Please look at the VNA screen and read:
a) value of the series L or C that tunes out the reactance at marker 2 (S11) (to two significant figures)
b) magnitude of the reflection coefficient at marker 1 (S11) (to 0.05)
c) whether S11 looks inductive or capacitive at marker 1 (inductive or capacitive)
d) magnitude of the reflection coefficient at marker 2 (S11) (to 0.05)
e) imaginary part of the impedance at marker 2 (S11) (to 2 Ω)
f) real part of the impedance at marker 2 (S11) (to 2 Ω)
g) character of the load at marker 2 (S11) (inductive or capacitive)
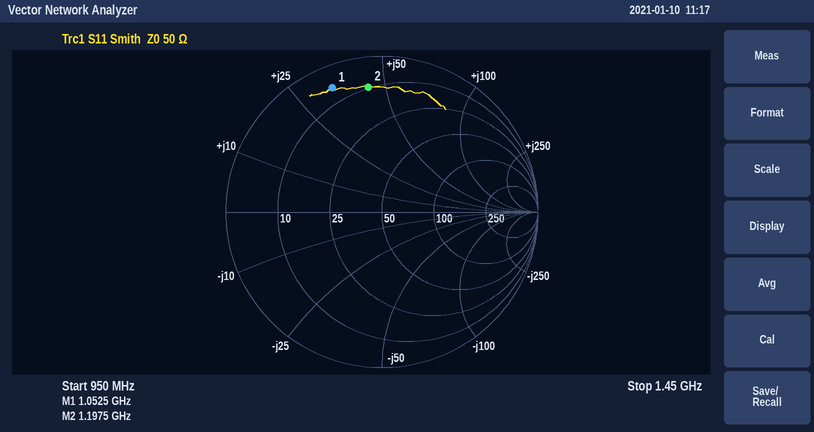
3.0 pF
0.85
inductive
0.80
+44 Ω
10 Ω
inductive
